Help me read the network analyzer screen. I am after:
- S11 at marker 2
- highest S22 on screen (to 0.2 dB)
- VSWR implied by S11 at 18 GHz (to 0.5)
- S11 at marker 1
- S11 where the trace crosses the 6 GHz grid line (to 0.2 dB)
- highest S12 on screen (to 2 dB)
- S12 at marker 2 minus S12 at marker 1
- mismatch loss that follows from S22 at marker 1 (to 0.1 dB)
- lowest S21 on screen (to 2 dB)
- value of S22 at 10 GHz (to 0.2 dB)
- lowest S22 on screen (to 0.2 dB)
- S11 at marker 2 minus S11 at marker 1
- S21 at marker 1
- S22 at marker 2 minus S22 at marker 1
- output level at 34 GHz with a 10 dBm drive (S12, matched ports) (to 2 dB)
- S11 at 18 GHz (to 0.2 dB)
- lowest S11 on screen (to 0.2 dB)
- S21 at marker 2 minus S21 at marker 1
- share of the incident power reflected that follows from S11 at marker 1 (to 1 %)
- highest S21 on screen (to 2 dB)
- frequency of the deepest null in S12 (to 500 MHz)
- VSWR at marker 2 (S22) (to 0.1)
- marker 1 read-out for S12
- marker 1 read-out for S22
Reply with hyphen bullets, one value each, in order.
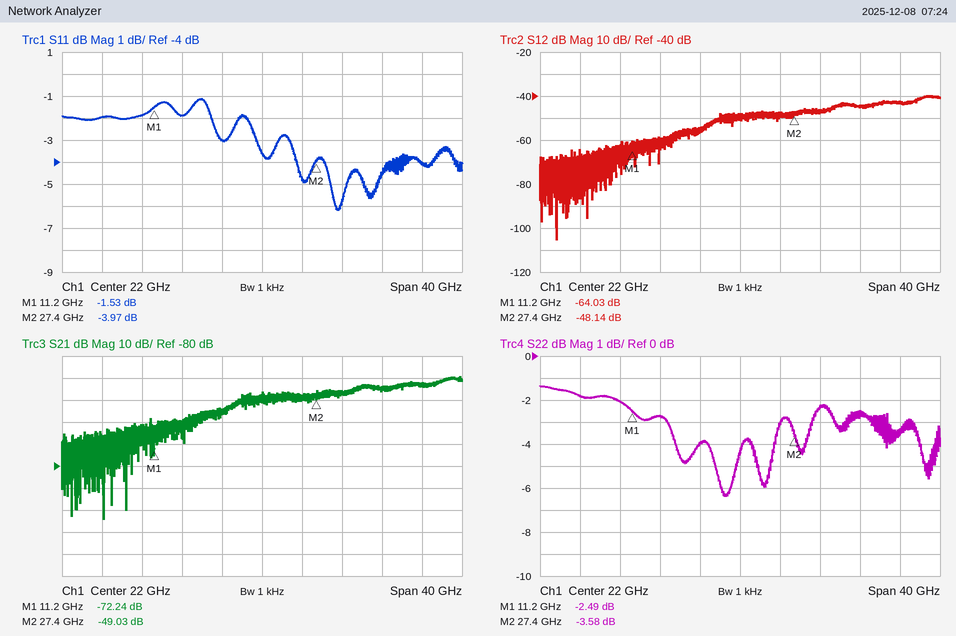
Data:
- -3.97 dB
- -1.4 dB
- 6.0
- -1.53 dB
- -2.0 dB
- -40 dB
- 15.89 dB
- 3.6 dB
- -104 dB
- -2.0 dB
- -6.4 dB
- -2.44 dB
- -72.24 dB
- -1.09 dB
- -34 dBm
- -3.0 dB
- -6.2 dB
- 23.21 dB
- 70 %
- -40 dB
- 3.5 GHz
- 4.9
- -64.03 dB
- -2.49 dB
